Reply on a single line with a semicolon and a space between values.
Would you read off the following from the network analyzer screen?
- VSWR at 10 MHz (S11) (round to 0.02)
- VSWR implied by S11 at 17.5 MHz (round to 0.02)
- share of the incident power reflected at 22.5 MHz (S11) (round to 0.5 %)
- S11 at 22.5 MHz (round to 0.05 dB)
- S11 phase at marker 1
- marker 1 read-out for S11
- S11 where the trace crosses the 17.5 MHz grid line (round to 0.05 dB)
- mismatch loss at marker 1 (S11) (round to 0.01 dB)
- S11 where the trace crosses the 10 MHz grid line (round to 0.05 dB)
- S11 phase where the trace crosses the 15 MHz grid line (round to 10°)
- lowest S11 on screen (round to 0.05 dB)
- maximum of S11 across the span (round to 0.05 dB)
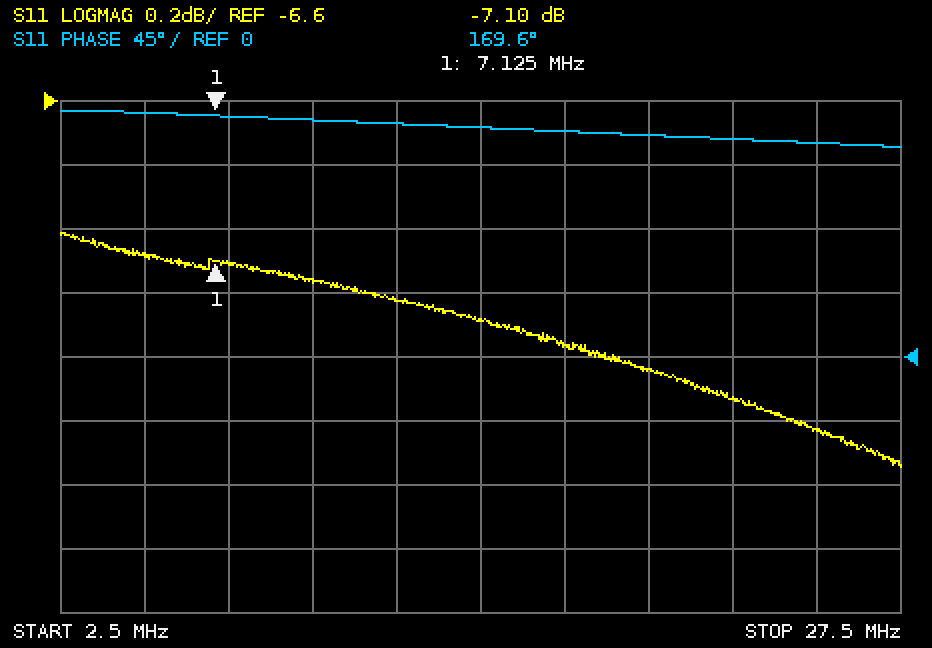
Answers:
2.56; 2.50; 17.5 %; -7.55 dB; 169.6°; -7.10 dB; -7.35 dB; 0.94 dB; -7.15 dB; 160°; -7.75 dB; -7.00 dB
